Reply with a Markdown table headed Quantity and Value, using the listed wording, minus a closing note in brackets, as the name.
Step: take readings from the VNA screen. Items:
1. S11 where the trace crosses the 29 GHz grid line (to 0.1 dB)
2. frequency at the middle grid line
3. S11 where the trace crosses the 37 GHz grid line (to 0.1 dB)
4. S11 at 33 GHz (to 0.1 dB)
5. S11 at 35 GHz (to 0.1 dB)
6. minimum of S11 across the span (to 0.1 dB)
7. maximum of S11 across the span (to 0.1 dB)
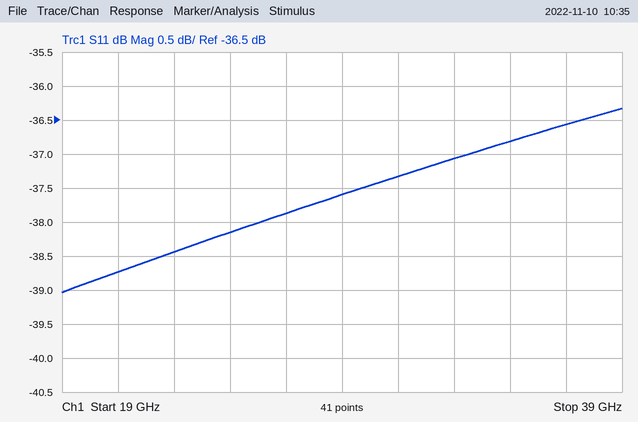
| Quantity | Value |
|---|---|
| S11 where the trace crosses the 29 GHz grid line | -37.6 dB |
| frequency at the middle grid line | 29 GHz |
| S11 where the trace crosses the 37 GHz grid line | -36.6 dB |
| S11 at 33 GHz | -37.1 dB |
| S11 at 35 GHz | -36.8 dB |
| minimum of S11 across the span | -39.0 dB |
| maximum of S11 across the span | -36.3 dB |
